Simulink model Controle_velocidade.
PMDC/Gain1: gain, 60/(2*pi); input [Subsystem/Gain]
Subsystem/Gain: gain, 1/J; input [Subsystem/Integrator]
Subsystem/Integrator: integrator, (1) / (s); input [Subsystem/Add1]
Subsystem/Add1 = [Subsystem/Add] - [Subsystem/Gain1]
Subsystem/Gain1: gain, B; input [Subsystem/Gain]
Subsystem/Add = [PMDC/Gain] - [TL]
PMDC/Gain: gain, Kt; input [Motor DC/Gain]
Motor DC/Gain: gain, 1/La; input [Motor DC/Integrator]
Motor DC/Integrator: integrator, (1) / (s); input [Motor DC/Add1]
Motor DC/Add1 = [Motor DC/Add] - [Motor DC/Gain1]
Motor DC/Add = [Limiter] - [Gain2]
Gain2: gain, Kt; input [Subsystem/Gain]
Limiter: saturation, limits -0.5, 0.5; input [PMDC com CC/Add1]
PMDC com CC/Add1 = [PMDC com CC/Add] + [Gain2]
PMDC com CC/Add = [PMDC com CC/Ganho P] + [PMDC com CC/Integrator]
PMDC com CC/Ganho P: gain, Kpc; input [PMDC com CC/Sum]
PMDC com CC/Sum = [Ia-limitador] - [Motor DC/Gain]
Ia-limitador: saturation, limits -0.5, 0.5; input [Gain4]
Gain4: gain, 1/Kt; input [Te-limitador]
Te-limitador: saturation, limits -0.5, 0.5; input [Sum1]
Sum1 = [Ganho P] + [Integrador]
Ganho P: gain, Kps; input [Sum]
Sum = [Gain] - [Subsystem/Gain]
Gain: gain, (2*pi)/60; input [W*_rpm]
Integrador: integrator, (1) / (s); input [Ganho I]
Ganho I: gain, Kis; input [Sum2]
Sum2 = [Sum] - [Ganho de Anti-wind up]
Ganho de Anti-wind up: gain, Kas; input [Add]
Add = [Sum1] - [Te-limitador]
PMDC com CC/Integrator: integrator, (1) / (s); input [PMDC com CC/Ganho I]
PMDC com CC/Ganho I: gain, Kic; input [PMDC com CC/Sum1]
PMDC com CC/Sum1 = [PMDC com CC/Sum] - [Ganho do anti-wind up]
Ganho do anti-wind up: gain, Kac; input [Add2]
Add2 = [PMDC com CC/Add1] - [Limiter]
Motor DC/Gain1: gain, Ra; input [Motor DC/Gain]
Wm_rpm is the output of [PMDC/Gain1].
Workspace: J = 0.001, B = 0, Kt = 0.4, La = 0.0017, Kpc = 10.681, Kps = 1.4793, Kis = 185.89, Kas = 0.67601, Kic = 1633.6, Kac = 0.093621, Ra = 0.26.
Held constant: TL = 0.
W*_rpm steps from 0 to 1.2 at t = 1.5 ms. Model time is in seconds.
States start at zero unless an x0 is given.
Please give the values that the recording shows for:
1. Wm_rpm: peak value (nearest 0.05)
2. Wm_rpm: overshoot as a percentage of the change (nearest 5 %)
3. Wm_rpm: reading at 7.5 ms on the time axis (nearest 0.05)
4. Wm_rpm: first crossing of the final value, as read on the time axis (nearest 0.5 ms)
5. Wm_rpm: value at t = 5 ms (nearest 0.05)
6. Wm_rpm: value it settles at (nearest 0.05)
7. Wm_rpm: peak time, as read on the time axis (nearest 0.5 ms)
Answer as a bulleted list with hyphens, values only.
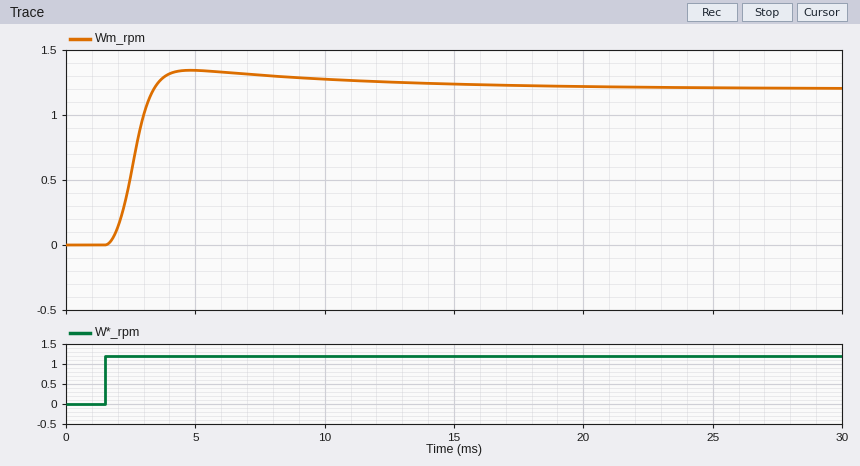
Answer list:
- 1.35
- 10 %
- 1.30
- 3.5 ms
- 1.35
- 1.20
- 5.0 ms
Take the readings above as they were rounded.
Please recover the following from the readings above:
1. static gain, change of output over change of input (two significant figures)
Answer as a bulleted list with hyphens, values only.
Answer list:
- 1.0
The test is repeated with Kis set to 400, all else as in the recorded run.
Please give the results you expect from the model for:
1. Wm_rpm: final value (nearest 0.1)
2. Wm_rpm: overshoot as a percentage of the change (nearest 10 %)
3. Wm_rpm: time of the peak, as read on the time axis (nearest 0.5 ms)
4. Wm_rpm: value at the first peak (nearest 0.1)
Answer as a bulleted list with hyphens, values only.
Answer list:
- 1.2
- 20 %
- 4.5 ms
- 1.5
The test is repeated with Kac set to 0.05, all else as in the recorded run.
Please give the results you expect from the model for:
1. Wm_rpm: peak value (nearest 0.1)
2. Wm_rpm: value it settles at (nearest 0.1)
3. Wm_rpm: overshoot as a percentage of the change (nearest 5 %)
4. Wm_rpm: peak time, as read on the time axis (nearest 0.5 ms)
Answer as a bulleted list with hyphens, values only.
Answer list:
- 1.4
- 1.2
- 15 %
- 4.5 ms
